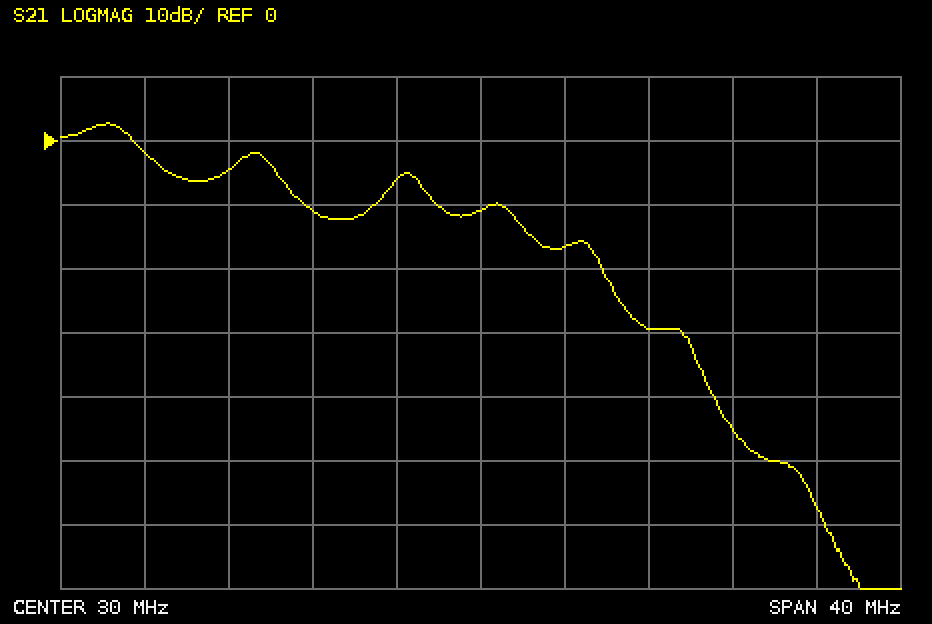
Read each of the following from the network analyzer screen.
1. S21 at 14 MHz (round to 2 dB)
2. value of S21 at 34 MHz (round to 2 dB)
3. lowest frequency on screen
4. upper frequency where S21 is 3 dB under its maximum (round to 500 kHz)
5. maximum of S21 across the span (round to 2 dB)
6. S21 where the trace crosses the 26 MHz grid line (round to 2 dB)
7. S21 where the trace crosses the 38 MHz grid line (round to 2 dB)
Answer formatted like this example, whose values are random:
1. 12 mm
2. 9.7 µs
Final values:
1. -2 dB
2. -16 dB
3. 10 MHz
4. 13.5 MHz
5. 2 dB
6. -6 dB
7. -30 dB
